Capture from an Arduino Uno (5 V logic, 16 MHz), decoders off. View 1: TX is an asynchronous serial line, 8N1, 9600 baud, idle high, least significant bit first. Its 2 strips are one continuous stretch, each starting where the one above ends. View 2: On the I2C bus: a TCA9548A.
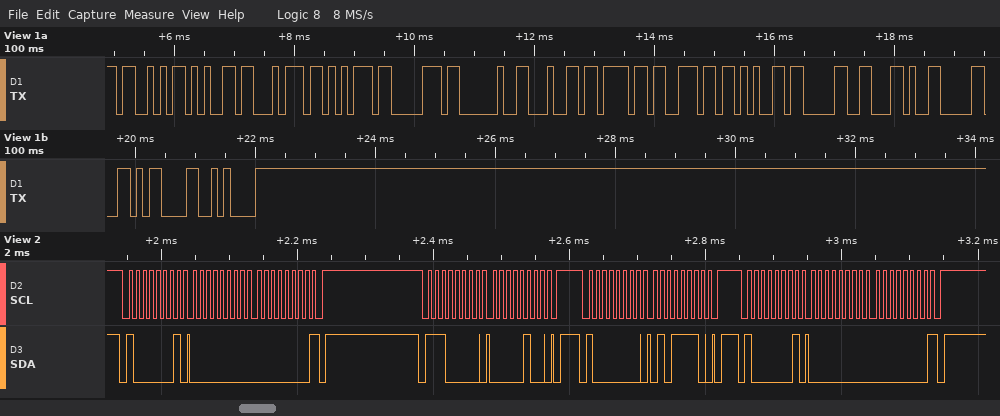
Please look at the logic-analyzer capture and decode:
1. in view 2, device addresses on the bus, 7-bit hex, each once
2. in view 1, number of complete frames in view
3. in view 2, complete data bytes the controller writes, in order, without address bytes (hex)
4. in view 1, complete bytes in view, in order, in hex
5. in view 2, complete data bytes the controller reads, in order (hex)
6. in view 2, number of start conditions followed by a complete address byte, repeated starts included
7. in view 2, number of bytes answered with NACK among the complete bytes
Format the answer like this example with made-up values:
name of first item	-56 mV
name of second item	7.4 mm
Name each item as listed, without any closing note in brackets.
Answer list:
in view 2, device addresses on the bus, 7-bit hex, each once	0x40 0x70
in view 1, number of complete frames in view	15
in view 2, complete data bytes the controller writes, in order, without address bytes	04 5E
in view 1, complete bytes in view, in order, in hex	0x53 0x65 0x74 0x75 0x70 0x20 0x64 0x6F 0x6E 0x65 0x30 0x2C 0x30 0x0D 0x0A
in view 2, complete data bytes the controller reads, in order	00 00 00 00
in view 2, number of start conditions followed by a complete address byte, repeated starts included	4
in view 2, number of bytes answered with NACK among the complete bytes	2
